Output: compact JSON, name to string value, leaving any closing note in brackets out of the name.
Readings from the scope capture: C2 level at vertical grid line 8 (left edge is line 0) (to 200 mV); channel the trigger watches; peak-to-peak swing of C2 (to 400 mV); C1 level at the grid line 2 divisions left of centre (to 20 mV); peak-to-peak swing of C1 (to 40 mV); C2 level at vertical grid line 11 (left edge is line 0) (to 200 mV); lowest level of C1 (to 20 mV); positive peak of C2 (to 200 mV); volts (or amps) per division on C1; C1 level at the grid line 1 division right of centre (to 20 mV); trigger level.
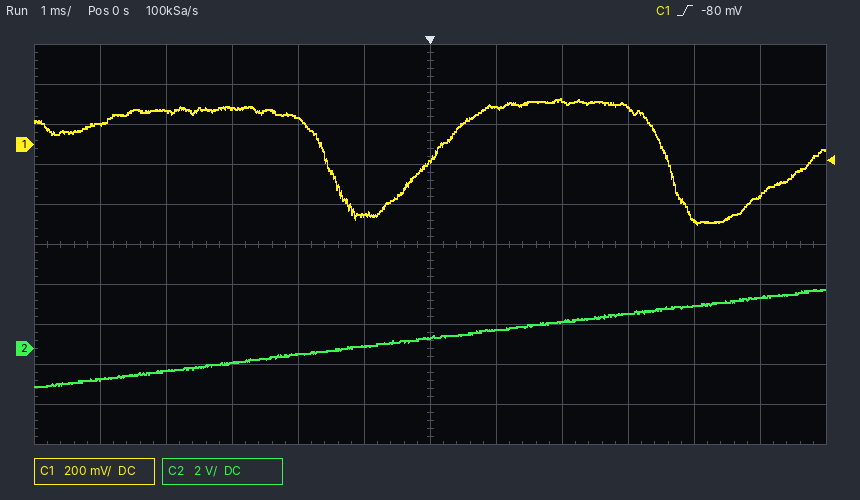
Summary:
{"C2 level at vertical grid line 8 (left edge is line 0)": "1.4 V", "channel the trigger watches": "C1", "peak-to-peak swing of C2": "4.8 V", "C1 level at the grid line 2 divisions left of centre": "140 mV", "peak-to-peak swing of C1": "640 mV", "C2 level at vertical grid line 11 (left edge is line 0)": "2.6 V", "lowest level of C1": "-400 mV", "positive peak of C2": "3.0 V", "volts (or amps) per division on C1": "200 mV", "C1 level at the grid line 1 division right of centre": "180 mV", "trigger level": "-80 mV"}
